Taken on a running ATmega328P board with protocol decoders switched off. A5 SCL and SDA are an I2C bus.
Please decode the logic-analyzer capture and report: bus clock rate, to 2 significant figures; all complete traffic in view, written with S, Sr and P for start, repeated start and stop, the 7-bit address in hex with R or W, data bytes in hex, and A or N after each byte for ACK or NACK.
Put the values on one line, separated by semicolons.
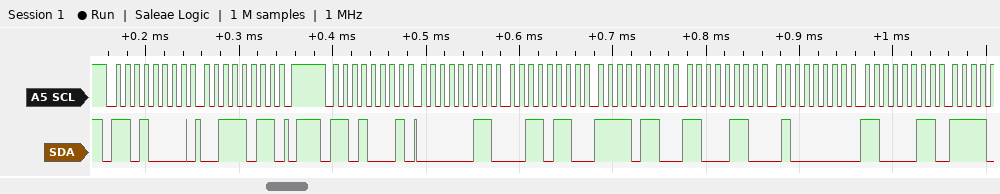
100 kHz; S 68W A 3B A P S 68R A 03 A 36 A F6 A C6 A 40 A C3 A
